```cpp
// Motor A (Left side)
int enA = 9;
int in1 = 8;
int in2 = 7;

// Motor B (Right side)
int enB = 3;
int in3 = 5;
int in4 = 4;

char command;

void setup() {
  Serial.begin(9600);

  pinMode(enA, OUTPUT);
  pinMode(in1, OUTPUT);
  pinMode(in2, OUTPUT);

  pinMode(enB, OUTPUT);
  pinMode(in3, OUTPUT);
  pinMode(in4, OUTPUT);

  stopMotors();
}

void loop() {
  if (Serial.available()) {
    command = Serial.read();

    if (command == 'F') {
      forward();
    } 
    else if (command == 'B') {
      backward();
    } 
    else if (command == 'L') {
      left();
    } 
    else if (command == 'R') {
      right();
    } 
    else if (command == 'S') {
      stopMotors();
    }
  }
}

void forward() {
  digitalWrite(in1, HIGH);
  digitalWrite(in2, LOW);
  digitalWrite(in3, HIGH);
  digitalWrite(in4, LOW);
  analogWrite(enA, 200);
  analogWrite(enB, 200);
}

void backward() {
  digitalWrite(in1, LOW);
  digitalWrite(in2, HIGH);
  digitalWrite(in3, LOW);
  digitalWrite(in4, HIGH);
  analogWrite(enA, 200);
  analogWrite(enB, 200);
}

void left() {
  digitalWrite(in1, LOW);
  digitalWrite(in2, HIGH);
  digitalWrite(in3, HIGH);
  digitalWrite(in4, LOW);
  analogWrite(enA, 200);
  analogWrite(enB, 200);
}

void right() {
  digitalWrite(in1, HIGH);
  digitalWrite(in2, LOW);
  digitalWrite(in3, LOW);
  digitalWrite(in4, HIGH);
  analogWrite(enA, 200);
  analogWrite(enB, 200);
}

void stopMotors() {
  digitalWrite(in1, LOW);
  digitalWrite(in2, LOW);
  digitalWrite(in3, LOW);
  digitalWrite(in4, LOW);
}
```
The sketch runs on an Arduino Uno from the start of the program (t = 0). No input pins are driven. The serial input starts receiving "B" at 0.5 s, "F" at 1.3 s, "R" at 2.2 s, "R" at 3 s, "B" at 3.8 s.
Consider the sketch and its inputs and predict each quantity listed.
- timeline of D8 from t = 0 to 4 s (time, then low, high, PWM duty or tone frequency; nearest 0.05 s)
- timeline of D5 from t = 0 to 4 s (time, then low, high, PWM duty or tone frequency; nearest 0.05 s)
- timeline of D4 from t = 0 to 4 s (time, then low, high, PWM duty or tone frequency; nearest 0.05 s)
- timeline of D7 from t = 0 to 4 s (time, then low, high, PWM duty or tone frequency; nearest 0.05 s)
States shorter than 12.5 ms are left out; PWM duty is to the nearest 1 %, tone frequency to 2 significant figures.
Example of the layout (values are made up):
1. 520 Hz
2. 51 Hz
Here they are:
1. 0 s low; 1.3 s high; 3.8 s low
2. 0 s low; 1.3 s high; 2.2 s low
3. 0 s low; 0.5 s high; 1.3 s low; 2.2 s high
4. 0 s low; 0.5 s high; 1.3 s low; 3.8 s high
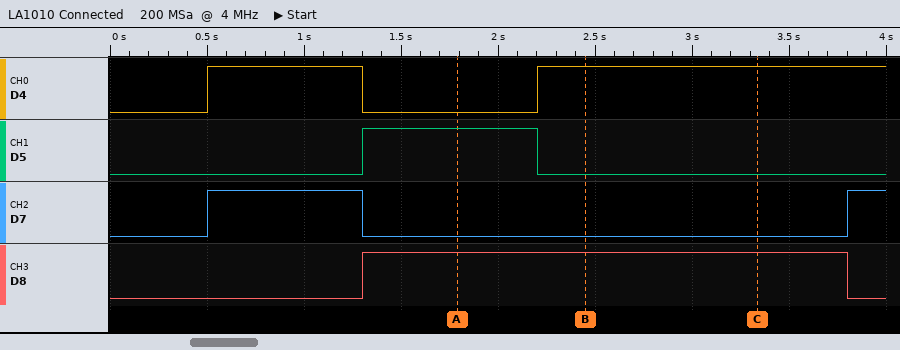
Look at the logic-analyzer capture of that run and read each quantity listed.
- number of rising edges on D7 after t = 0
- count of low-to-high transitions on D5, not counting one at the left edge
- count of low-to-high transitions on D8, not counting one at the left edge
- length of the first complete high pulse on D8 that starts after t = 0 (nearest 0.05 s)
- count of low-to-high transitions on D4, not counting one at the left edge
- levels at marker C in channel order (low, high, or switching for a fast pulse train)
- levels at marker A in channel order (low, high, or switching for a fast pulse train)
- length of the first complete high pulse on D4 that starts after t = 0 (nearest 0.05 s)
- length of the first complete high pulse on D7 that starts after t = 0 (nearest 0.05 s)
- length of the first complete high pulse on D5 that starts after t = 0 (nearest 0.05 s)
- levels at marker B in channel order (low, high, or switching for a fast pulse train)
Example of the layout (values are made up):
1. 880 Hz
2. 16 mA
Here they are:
1. 2
2. 1
3. 1
4. 2.50 s
5. 2
6. D4 high, D5 low, D7 low, D8 high
7. D4 low, D5 high, D7 low, D8 high
8. 0.80 s
9. 0.80 s
10. 0.90 s
11. D4 high, D5 low, D7 low, D8 high
